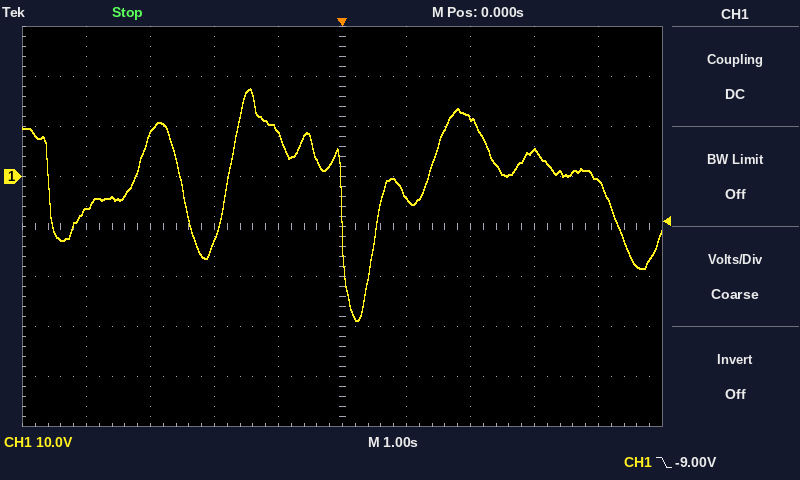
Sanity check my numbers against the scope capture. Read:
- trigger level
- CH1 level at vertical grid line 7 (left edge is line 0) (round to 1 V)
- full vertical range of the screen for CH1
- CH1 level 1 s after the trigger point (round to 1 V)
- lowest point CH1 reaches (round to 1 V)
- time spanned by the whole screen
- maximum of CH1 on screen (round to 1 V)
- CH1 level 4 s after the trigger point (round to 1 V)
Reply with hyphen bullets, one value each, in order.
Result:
- -9.00 V
- 12 V
- 80 V
- -4 V
- -29 V
- 10 s
- 18 V
- -1 V
